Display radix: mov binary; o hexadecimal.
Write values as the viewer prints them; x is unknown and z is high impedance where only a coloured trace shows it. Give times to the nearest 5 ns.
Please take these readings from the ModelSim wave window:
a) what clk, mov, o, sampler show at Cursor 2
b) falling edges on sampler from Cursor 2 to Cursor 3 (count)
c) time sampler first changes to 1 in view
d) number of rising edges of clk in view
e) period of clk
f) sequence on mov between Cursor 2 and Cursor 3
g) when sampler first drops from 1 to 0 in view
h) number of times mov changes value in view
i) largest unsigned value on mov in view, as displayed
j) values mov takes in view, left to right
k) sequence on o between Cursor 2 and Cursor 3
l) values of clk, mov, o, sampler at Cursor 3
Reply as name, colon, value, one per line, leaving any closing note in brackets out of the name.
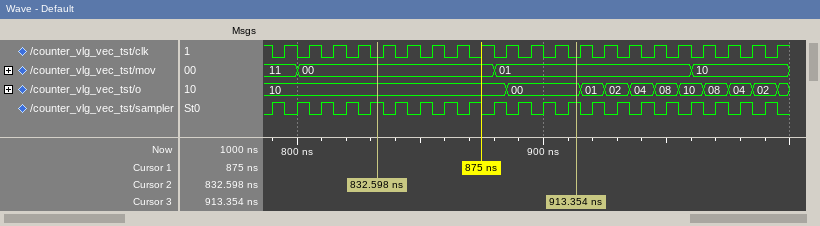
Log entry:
what clk, mov, o, sampler show at Cursor 2: clk=0, mov=00, o=10, sampler=1
falling edges on sampler from Cursor 2 to Cursor 3: 8
time sampler first changes to 1 in view: 790 ns
number of rising edges of clk in view: 21
period of clk: 10 ns
sequence on mov between Cursor 2 and Cursor 3: 00, 01
when sampler first drops from 1 to 0 in view: 795 ns
number of times mov changes value in view: 3
largest unsigned value on mov in view, as displayed: 11
values mov takes in view, left to right: 11, 00, 01, 10
sequence on o between Cursor 2 and Cursor 3: 10, 00
values of clk, mov, o, sampler at Cursor 3: clk=0, mov=01, o=00, sampler=1
